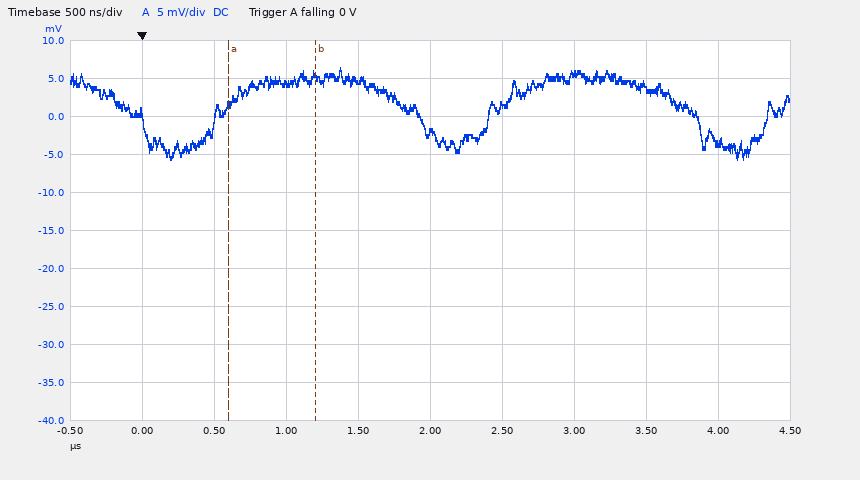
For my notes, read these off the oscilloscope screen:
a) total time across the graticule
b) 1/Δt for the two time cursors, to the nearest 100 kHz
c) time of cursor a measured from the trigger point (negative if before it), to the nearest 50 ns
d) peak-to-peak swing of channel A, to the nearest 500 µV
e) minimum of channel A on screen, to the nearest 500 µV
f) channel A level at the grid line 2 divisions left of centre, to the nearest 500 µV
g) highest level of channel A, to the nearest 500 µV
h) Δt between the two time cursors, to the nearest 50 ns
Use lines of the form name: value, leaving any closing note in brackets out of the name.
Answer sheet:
total time across the graticule: 5 µs
1/Δt for the two time cursors, to the nearest 100 kHz: 1.7 MHz
time of cursor a measured from the trigger point (negative if before it), to the nearest 50 ns: +600 ns
peak-to-peak swing of channel A, to the nearest 500 µV: 12.0 mV
minimum of channel A on screen, to the nearest 500 µV: -5.5 mV
channel A level at the grid line 2 divisions left of centre, to the nearest 500 µV: 4.5 mV
highest level of channel A, to the nearest 500 µV: 6.5 mV
Δt between the two time cursors, to the nearest 50 ns: 600 ns
